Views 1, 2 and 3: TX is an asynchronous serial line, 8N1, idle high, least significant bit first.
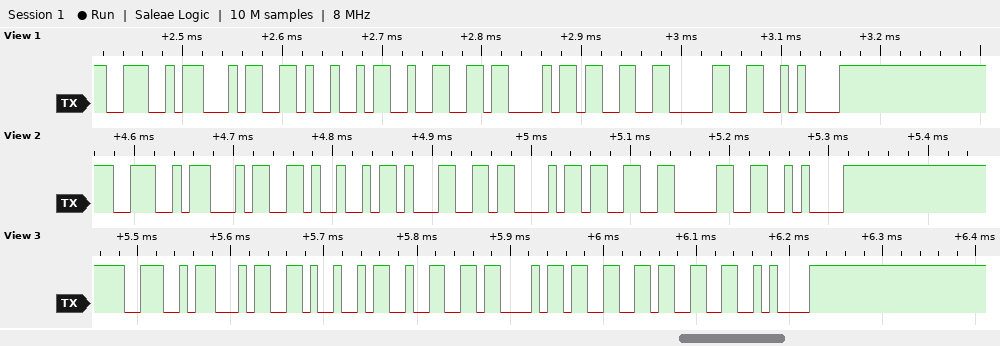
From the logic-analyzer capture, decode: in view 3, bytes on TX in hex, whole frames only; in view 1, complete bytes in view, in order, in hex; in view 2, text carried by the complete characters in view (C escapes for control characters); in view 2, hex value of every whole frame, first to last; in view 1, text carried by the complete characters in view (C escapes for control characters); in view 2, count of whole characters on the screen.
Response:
4E 34 49 32 43 33 33 0A
0x4E 0x34 0x49 0x32 0x43 0x33 0x30 0x0A
"N4I1C30\n"
0x4E 0x34 0x49 0x31 0x43 0x33 0x30 0x0A
"N4I2C30\n"
8
